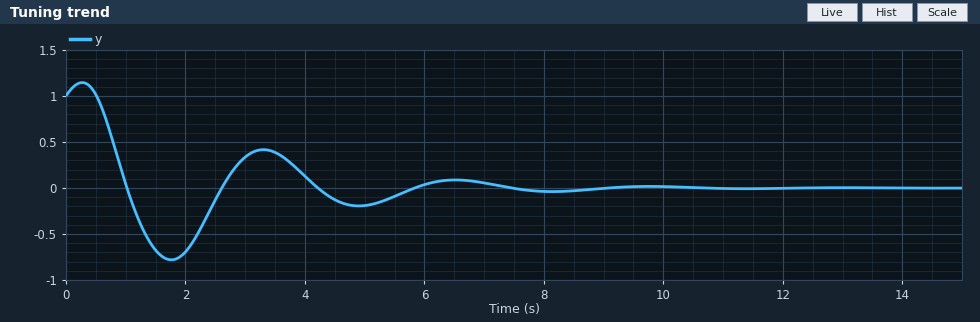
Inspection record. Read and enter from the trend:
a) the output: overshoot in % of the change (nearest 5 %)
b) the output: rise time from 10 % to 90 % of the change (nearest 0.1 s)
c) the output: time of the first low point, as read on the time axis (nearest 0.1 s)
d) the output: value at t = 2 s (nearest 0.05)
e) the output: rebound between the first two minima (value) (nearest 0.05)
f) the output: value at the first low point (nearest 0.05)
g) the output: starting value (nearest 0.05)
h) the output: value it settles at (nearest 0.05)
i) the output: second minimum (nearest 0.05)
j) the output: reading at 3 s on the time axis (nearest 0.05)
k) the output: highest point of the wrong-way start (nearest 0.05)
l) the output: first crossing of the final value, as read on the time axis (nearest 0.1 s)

80 %
0.4 s
1.8 s
-0.70
0.40
-0.80
1.00
0.00
-0.20
0.35
1.15
1.0 s
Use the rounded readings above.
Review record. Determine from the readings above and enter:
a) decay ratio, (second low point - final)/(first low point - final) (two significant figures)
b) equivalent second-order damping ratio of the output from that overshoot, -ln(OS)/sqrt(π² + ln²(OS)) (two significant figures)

0.25
0.071
